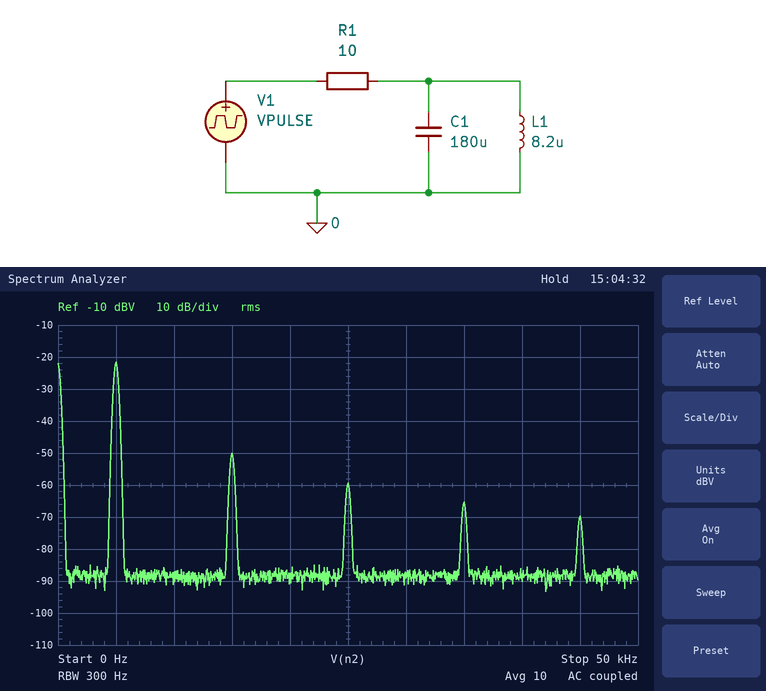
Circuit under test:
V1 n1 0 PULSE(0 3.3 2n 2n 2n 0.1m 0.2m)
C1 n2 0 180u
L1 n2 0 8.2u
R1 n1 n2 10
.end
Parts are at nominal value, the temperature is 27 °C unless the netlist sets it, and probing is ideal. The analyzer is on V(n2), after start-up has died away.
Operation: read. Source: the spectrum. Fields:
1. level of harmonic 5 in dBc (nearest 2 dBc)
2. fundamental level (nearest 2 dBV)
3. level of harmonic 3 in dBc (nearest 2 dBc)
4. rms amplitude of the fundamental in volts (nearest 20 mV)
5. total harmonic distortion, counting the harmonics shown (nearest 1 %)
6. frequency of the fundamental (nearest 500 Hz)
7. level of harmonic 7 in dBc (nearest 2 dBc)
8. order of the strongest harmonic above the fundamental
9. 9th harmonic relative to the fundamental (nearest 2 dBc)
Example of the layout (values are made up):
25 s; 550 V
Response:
-38 dBc; -22 dBV; -28 dBc; 80 mV; 4 %; 5.0 kHz; -44 dBc; 3; -48 dBc
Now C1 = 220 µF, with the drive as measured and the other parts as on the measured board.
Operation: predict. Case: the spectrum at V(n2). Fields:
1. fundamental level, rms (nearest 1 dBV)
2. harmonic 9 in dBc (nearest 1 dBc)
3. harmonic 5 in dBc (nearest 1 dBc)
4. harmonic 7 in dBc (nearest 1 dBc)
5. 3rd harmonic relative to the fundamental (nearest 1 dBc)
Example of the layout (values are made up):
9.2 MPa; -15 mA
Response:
-26 dBV; -45 dBc; -35 dBc; -41 dBc; -26 dBc
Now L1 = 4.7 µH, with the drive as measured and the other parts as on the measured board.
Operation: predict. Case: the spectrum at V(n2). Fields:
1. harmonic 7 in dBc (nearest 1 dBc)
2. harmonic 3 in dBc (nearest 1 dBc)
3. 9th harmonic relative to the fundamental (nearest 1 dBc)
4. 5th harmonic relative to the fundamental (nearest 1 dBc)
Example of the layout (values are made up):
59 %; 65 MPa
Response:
-48 dBc; -32 dBc; -52 dBc; -42 dBc
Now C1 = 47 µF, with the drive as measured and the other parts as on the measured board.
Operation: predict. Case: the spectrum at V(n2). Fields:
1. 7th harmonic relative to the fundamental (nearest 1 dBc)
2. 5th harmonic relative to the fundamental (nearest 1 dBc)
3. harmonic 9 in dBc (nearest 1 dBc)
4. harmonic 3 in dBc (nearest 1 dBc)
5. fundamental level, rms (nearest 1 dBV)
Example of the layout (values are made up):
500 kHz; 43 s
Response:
-29 dBc; -23 dBc; -34 dBc; -12 dBc; -24 dBV
